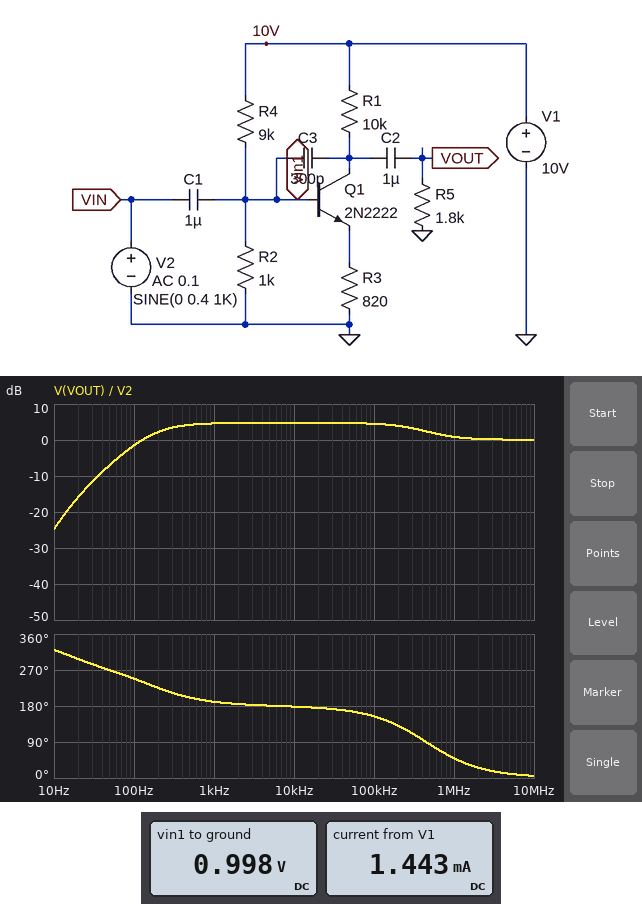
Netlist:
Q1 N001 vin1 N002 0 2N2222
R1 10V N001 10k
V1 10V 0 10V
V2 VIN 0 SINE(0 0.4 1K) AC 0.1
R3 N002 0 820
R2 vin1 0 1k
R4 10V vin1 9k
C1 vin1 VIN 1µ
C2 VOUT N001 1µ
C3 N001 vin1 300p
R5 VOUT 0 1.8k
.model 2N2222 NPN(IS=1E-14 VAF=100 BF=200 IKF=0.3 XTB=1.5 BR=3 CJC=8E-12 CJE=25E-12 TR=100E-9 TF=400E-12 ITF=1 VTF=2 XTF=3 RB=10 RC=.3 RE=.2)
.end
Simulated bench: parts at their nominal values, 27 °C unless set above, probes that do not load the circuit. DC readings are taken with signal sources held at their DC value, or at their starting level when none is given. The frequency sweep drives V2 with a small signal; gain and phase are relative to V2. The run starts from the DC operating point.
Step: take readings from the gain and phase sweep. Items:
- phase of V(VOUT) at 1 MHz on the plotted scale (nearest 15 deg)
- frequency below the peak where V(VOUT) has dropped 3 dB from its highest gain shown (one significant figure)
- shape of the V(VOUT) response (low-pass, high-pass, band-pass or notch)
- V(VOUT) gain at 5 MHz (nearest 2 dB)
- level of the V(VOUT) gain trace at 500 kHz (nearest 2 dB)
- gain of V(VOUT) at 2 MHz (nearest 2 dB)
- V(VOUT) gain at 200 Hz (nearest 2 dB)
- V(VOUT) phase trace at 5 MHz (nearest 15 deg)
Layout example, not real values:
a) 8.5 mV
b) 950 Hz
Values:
a) 45 deg
b) 200 Hz
c) high-pass
d) 0 dB
e) 2 dB
f) 0 dB
g) 2 dB
h) 15 deg
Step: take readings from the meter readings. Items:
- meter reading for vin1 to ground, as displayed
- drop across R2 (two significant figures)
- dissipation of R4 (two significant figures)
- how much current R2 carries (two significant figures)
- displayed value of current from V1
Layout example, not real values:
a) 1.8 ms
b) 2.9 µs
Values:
a) 0.998 V
b) 1.0 V
c) 9.0 mW
d) 1.0 mA
e) 1.443 mA
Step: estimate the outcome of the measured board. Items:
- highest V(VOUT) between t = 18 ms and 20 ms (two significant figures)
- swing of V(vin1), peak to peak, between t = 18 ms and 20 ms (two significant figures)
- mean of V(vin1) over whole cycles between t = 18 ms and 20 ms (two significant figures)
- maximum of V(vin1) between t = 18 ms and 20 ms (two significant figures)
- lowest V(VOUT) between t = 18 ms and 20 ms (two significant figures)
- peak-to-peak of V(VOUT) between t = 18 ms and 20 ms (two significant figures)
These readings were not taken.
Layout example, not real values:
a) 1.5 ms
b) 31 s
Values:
a) 630 mV
b) 790 mV
c) 1.0 V
d) 1.4 V
e) -680 mV
f) 1.3 V
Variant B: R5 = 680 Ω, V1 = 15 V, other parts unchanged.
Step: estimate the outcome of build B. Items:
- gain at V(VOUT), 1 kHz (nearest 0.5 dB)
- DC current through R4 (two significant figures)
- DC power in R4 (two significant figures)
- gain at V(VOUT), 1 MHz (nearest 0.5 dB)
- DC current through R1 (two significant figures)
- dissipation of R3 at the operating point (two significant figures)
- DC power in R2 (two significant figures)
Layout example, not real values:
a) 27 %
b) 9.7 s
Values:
a) -2.5 dB
b) 1.5 mA
c) 20 mW
d) -1.0 dB
e) 1.0 mA
f) 860 µW
g) 2.2 mW
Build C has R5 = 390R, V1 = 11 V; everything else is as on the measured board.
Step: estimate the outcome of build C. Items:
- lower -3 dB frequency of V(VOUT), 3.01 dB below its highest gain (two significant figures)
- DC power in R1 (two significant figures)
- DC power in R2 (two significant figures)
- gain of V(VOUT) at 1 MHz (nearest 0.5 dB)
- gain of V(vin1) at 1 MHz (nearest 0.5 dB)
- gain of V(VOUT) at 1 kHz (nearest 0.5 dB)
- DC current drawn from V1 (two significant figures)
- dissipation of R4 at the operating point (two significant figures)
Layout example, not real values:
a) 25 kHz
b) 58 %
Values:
a) 1.1 MHz
b) 3.1 mW
c) 1.2 mW
d) -3.5 dB
e) 0 dB
f) -7.5 dB
g) 1.7 mA
h) 11 mW
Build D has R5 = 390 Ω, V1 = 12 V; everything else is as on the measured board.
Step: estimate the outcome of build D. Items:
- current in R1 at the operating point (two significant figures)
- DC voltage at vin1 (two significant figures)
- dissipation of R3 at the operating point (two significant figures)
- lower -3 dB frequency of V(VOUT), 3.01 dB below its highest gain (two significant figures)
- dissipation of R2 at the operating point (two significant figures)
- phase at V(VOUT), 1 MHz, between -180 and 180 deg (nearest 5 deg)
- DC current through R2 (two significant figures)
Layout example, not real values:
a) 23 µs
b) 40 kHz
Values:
a) 670 µA
b) 1.2 V
c) 370 µW
d) 1.1 MHz
e) 1.4 mW
f) 85 deg
g) 1.2 mA
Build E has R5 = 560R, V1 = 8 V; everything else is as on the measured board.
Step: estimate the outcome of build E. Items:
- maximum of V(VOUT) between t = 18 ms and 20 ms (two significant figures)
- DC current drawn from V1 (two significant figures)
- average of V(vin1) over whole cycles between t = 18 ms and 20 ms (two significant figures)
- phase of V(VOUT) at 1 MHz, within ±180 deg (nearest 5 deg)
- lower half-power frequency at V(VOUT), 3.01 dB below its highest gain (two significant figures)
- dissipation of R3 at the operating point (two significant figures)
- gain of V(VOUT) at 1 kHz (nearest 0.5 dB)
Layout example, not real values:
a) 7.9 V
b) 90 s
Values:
a) 140 mV
b) 1.0 mA
c) 800 mV
d) 75 deg
e) 600 kHz
f) 41 µW
g) -5.0 dB
